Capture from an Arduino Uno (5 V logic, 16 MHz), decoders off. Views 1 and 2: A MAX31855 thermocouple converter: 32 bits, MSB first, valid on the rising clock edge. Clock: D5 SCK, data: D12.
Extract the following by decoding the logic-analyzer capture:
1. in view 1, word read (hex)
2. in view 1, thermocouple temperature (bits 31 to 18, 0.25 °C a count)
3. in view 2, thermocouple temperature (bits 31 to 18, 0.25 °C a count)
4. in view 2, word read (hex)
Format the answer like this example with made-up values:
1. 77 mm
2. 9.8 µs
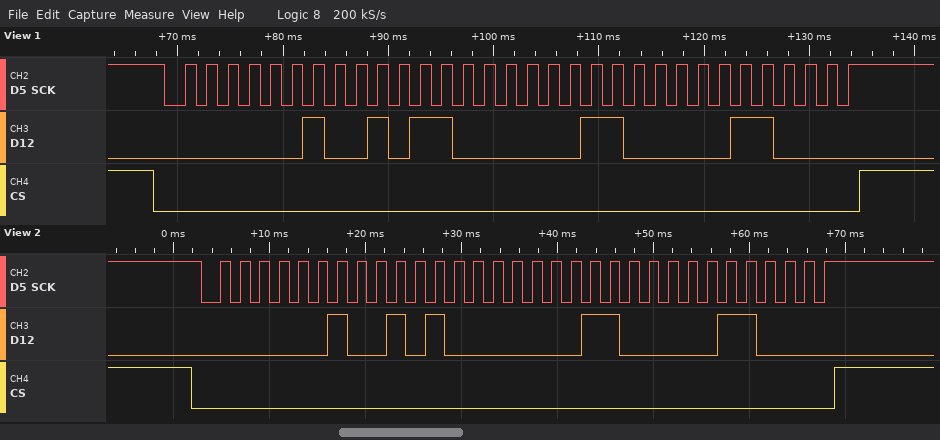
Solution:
1. 0x02581830
2. 37.50 °C
3. 37.00 °C
4. 0x02501830
